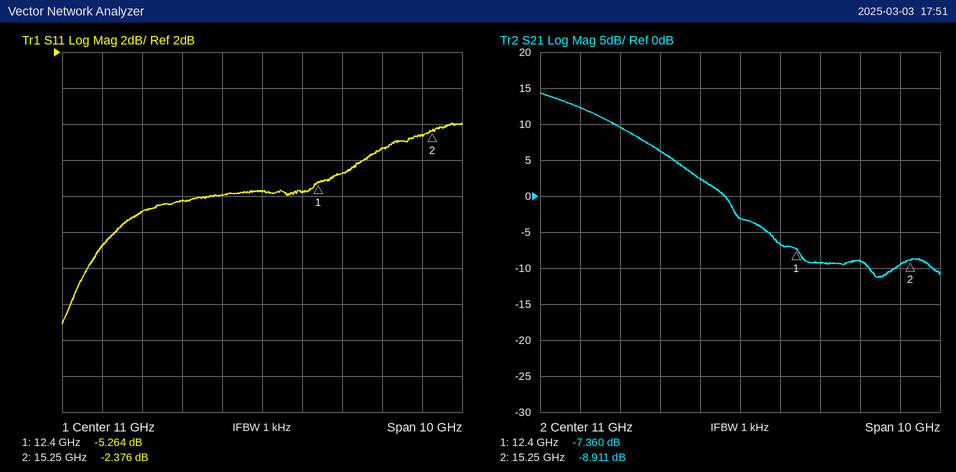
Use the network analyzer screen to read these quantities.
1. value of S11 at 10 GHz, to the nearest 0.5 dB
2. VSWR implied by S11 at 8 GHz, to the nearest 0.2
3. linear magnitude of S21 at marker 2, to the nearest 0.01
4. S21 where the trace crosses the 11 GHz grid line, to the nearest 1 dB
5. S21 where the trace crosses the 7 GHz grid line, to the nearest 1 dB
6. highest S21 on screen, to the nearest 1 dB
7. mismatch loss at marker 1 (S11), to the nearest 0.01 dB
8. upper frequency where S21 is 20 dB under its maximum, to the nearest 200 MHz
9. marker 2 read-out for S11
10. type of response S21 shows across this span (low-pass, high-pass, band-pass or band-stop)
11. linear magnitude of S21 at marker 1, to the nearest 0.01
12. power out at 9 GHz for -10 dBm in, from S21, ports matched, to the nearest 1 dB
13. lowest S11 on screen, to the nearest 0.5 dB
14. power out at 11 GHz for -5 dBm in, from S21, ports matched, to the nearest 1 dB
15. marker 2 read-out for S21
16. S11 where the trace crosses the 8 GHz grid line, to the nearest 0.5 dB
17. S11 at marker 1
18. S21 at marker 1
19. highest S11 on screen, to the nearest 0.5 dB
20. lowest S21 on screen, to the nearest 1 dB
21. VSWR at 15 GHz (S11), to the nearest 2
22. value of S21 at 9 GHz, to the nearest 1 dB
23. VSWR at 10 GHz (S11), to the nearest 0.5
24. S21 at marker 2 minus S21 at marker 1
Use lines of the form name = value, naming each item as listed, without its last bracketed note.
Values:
value of S11 at 10 GHz, to the nearest 0.5 dB = -6.0 dB
VSWR implied by S11 at 8 GHz, to the nearest 0.2 = 2.6
linear magnitude of S21 at marker 2, to the nearest 0.01 = 0.36
S21 where the trace crosses the 11 GHz grid line, to the nearest 1 dB = -3 dB
S21 where the trace crosses the 7 GHz grid line, to the nearest 1 dB = 12 dB
highest S21 on screen, to the nearest 1 dB = 14 dB
mismatch loss at marker 1 (S11), to the nearest 0.01 dB = 1.53 dB
upper frequency where S21 is 20 dB under its maximum, to the nearest 200 MHz = 11.8 GHz
marker 2 read-out for S11 = -2.376 dB
type of response S21 shows across this span = low-pass
linear magnitude of S21 at marker 1, to the nearest 0.01 = 0.43
power out at 9 GHz for -10 dBm in, from S21, ports matched, to the nearest 1 dB = -4 dBm
lowest S11 on screen, to the nearest 0.5 dB = -13.0 dB
power out at 11 GHz for -5 dBm in, from S21, ports matched, to the nearest 1 dB = -8 dBm
marker 2 read-out for S21 = -8.911 dB
S11 where the trace crosses the 8 GHz grid line, to the nearest 0.5 dB = -7.0 dB
S11 at marker 1 = -5.264 dB
S21 at marker 1 = -7.360 dB
highest S11 on screen, to the nearest 0.5 dB = -2.0 dB
lowest S21 on screen, to the nearest 1 dB = -11 dB
VSWR at 15 GHz (S11), to the nearest 2 = 6
value of S21 at 9 GHz, to the nearest 1 dB = 6 dB
VSWR at 10 GHz (S11), to the nearest 0.5 = 3.0
S21 at marker 2 minus S21 at marker 1 = -1.551 dB
